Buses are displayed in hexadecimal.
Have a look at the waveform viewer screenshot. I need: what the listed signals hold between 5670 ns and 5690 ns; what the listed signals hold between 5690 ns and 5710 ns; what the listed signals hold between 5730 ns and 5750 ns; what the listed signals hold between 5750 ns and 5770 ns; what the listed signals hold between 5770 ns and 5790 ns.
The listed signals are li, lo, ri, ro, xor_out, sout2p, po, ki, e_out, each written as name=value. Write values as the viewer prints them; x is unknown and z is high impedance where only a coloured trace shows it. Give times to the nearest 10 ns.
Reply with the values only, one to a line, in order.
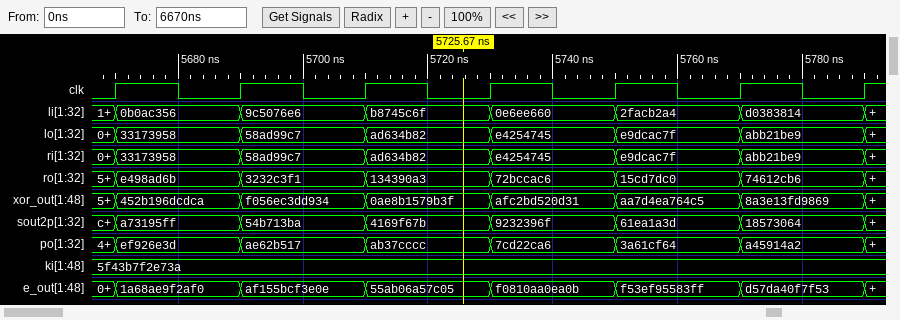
li=0b0ac356, lo=33173958, ri=33173958, ro=e498ad6b, xor_out=452b196dcdca, sout2p=a73195ff, po=ef926e3d, ki=5f43b7f2e73a, e_out=1a68ae9f2af0
li=9c5076e6, lo=58ad99c7, ri=58ad99c7, ro=3232c3f1, xor_out=f056ec3dd934, sout2p=54b713ba, po=ae62b517, ki=5f43b7f2e73a, e_out=af155bcf3e0e
li=0e6ee660, lo=e4254745, ri=e4254745, ro=72bccac6, xor_out=afc2bd520d31, sout2p=9232396f, po=7cd22ca6, ki=5f43b7f2e73a, e_out=f0810aa0ea0b
li=2facb2a4, lo=e9dcac7f, ri=e9dcac7f, ro=15cd7dc0, xor_out=aa7d4ea764c5, sout2p=61ea1a3d, po=3a61cf64, ki=5f43b7f2e73a, e_out=f53ef95583ff
li=d0383814, lo=abb21be9, ri=abb21be9, ro=74612cb6, xor_out=8a3e13fd9869, sout2p=18573064, po=a45914a2, ki=5f43b7f2e73a, e_out=d57da40f7f53
